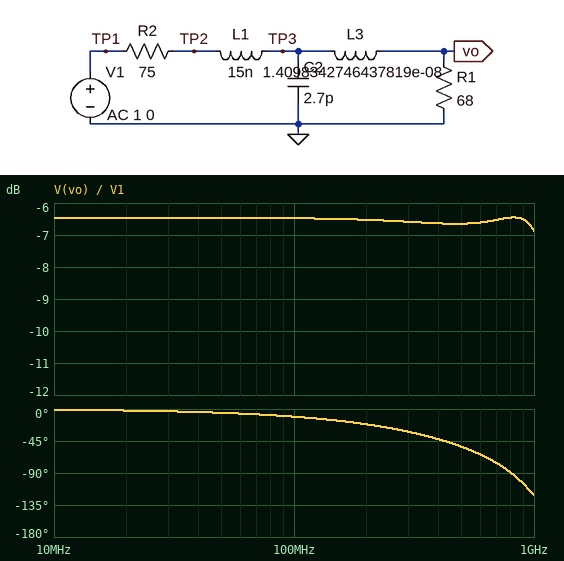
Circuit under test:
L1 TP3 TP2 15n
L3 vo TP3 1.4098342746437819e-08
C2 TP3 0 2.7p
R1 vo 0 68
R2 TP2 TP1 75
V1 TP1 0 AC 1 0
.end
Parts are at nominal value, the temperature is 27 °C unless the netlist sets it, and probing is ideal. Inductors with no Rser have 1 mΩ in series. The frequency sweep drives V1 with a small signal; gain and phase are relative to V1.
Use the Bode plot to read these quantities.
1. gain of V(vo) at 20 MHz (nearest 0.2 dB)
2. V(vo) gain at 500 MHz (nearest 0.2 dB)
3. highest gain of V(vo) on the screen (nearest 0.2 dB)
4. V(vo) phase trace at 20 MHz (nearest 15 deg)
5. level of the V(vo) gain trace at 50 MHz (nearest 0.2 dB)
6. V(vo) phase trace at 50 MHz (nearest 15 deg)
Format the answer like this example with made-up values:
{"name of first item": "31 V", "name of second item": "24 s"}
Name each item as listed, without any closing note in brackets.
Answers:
{"gain of V(vo) at 20 MHz": "-6.4 dB", "V(vo) gain at 500 MHz": "-6.6 dB", "highest gain of V(vo) on the screen": "-6.4 dB", "V(vo) phase trace at 20 MHz": "0 deg", "level of the V(vo) gain trace at 50 MHz": "-6.4 dB", "V(vo) phase trace at 50 MHz": "0 deg"}
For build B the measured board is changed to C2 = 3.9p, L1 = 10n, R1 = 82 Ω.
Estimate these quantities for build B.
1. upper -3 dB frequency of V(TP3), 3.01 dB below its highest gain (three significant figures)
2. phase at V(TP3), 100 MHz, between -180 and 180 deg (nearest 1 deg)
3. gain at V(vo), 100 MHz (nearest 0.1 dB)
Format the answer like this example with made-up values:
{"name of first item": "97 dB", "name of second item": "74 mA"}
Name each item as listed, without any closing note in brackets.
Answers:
{"upper -3 dB frequency of V(TP3), 3.01 dB below its highest gain": "1.24 GHz", "phase at V(TP3), 100 MHz, between -180 and 180 deg": "-5 deg", "gain at V(vo), 100 MHz": "-5.6 dB"}
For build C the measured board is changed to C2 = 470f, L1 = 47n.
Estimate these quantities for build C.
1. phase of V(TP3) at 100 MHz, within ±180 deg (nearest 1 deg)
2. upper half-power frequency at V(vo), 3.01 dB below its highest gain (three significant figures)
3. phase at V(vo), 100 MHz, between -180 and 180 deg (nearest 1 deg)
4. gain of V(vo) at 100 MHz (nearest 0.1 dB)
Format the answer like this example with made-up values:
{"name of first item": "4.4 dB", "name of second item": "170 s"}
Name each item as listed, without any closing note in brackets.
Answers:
{"phase of V(TP3) at 100 MHz, within ±180 deg": "-8 deg", "upper half-power frequency at V(vo), 3.01 dB below its highest gain": "400 MHz", "phase at V(vo), 100 MHz, between -180 and 180 deg": "-16 deg", "gain of V(vo) at 100 MHz": "-6.7 dB"}
